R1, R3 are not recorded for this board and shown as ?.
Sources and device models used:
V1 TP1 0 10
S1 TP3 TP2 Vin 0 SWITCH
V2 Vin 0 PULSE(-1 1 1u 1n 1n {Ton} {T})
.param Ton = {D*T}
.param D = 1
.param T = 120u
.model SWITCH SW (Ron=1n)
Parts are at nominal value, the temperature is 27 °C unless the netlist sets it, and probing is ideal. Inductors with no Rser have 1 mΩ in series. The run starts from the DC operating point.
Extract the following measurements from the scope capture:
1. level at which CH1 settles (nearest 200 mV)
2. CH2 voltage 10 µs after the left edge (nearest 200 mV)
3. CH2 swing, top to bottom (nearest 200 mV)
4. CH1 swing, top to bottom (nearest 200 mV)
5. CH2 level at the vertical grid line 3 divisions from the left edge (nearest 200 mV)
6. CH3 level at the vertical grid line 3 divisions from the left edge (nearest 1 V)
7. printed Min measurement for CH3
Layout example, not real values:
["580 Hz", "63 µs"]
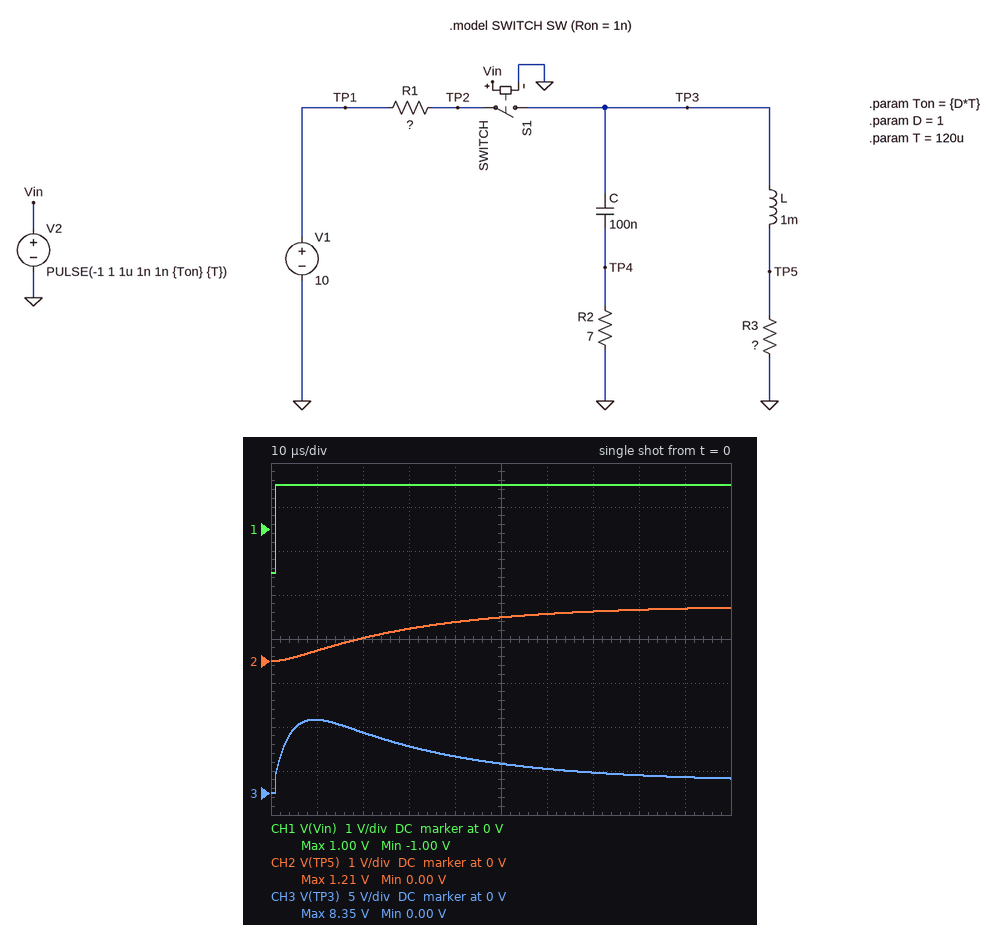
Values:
["1.0 V", "200 mV", "1.2 V", "2.0 V", "800 mV", "5 V", "0.00 V"]
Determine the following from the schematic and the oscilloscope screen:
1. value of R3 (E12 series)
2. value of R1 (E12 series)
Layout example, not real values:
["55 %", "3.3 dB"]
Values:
["3.9 Ω", "27 Ω"]
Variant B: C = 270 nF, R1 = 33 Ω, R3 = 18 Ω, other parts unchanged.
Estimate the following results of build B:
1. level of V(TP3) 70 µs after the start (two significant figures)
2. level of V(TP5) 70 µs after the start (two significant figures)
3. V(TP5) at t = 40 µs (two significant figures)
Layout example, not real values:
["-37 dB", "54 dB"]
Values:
["3.7 V", "3.5 V", "3.0 V"]
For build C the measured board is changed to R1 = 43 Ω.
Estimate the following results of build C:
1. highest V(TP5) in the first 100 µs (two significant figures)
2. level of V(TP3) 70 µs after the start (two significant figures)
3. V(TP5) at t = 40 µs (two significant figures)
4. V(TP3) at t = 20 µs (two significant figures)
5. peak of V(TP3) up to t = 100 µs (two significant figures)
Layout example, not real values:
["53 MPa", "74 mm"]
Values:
["830 mV", "1.1 V", "720 mV", "6.0 V", "7.4 V"]
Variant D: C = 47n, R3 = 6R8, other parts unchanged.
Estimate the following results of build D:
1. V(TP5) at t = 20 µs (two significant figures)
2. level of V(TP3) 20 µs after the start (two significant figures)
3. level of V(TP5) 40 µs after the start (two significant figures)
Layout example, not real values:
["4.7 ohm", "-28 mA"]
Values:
["930 mV", "6.5 V", "1.5 V"]
